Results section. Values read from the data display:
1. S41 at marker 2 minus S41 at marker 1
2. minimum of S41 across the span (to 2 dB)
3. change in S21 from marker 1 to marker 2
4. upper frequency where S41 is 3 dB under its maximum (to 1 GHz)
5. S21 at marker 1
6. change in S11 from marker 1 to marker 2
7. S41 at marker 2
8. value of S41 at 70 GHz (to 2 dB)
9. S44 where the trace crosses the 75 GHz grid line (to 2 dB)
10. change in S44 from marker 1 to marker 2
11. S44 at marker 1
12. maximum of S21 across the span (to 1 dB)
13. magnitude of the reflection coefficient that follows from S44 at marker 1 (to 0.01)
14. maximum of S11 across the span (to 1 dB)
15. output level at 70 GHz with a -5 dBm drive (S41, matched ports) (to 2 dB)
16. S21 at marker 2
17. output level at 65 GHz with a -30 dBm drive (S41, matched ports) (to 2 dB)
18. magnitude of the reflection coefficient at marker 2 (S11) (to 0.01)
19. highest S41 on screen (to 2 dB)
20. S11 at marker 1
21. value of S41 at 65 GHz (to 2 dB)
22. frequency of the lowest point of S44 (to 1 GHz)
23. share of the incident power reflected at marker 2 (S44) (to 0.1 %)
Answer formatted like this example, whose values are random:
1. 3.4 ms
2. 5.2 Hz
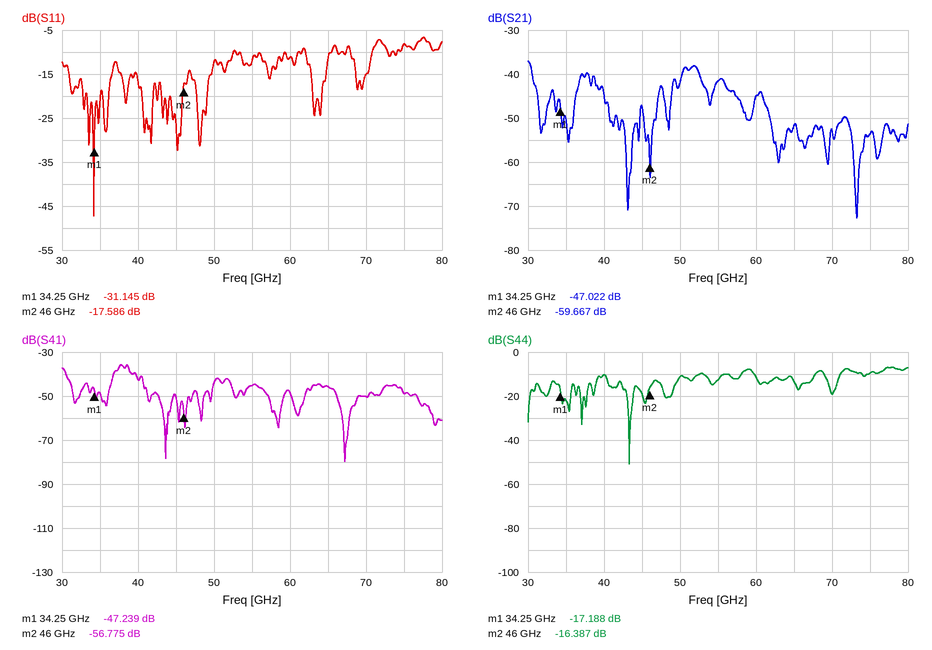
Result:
1. -9.536 dB
2. -80 dB
3. -12.645 dB
4. 39 GHz
5. -47.022 dB
6. 13.559 dB
7. -56.775 dB
8. -50 dB
9. -10 dB
10. 0.801 dB
11. -17.188 dB
12. -37 dB
13. 0.14
14. -7 dB
15. -56 dBm
16. -59.667 dB
17. -76 dBm
18. 0.13
19. -36 dB
20. -31.145 dB
21. -46 dB
22. 43 GHz
23. 2.3 %
